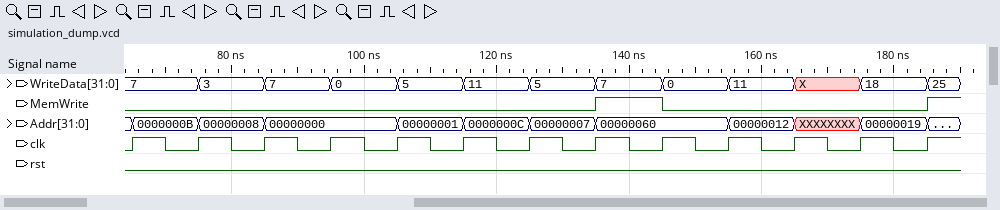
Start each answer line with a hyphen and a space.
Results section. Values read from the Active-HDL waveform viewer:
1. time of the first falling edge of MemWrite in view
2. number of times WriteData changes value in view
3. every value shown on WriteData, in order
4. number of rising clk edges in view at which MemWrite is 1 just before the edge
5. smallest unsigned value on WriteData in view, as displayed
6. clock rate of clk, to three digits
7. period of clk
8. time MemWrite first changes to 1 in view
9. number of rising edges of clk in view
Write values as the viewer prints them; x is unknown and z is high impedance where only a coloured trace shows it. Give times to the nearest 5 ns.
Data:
- 145 ns
- 12
- 7, 3, 7, 0, 5, 11, 5, 7, 0, 11, X, 18, 25
- 1
- 0
- 100 MHz
- 10 ns
- 135 ns
- 13
